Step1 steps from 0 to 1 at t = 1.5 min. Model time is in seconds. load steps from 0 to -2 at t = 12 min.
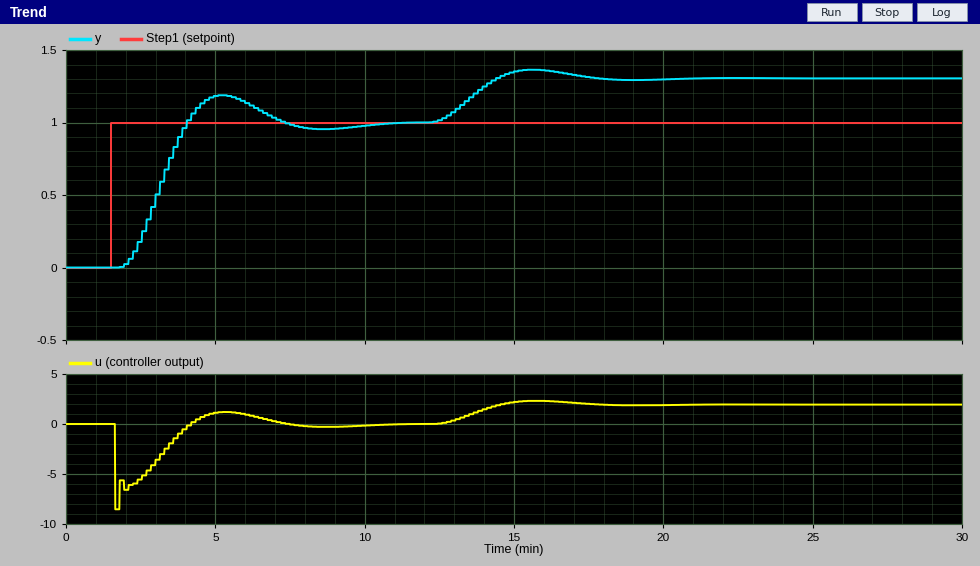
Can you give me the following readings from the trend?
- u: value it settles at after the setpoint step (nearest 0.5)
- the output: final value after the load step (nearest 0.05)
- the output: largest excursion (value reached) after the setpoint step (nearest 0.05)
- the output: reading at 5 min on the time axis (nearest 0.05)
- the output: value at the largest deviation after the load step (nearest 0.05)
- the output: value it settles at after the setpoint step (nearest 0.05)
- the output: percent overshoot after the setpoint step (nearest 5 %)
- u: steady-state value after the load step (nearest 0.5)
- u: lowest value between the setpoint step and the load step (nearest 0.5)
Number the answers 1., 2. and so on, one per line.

1. 0.0
2. 1.30
3. 1.20
4. 1.20
5. 1.35
6. 1.00
7. 20 %
8. 2.0
9. -8.5
